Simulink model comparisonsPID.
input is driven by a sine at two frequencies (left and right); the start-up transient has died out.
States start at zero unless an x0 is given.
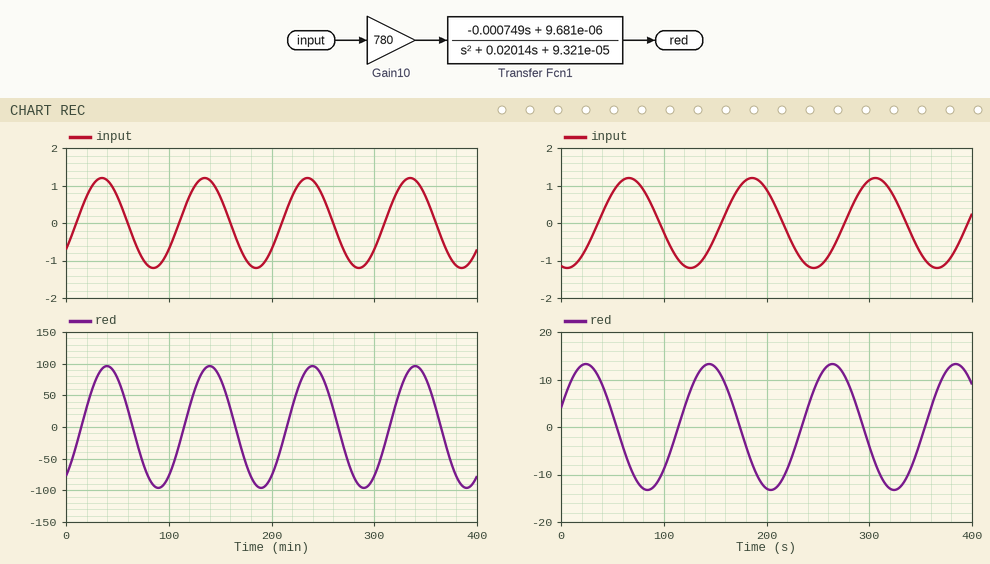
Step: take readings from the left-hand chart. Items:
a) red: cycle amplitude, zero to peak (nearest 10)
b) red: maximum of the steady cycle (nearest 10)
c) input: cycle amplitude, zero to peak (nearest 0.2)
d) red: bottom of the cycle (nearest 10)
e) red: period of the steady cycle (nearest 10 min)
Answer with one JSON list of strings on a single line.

["100", "100", "1.2", "-100", "100 min"]
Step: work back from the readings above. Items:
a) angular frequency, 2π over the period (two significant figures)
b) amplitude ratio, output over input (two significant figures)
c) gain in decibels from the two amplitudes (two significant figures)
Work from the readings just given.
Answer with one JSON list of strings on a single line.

["0.063 rad/min", "83", "38 dB"]
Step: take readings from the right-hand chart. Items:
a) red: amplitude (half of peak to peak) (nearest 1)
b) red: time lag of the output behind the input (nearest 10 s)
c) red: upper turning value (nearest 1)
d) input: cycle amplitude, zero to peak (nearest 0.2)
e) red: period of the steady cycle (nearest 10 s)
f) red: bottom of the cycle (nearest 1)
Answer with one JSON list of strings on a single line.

["13", "80 s", "13", "1.2", "120 s", "-13"]
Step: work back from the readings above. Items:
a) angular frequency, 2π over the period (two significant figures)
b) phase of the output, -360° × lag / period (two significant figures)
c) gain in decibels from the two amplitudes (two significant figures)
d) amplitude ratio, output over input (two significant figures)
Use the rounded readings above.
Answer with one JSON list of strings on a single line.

["0.052 rad/s", "-240°", "21 dB", "11"]
